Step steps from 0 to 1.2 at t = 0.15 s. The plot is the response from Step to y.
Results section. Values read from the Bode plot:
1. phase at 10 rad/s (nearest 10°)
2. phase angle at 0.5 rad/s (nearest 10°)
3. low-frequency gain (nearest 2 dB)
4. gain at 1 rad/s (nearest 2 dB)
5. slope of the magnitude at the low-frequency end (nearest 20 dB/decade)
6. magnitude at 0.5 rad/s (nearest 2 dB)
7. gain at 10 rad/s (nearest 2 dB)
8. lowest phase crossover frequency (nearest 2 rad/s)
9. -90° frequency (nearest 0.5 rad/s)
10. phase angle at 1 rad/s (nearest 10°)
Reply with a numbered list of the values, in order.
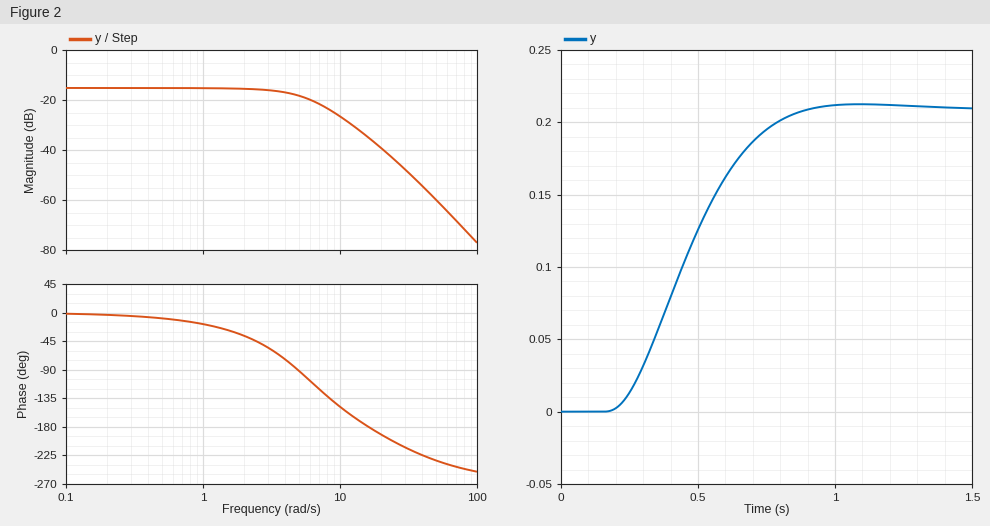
1. -150°
2. -10°
3. -16 dB
4. -16 dB
5. 0 dB/decade
6. -16 dB
7. -26 dB
8. 16 rad/s
9. 5.0 rad/s
10. -20°
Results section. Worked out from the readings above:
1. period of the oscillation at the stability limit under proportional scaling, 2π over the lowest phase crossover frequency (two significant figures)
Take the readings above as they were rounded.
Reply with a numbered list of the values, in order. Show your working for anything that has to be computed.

1. 2π / 16 = 0.39 s
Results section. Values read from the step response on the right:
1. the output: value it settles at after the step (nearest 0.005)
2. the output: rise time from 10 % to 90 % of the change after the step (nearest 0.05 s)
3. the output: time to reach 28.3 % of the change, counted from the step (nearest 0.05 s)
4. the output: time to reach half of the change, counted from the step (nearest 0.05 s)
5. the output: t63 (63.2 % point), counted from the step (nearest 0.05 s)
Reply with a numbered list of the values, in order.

1. 0.210
2. 0.45 s
3. 0.20 s
4. 0.30 s
5. 0.35 s
